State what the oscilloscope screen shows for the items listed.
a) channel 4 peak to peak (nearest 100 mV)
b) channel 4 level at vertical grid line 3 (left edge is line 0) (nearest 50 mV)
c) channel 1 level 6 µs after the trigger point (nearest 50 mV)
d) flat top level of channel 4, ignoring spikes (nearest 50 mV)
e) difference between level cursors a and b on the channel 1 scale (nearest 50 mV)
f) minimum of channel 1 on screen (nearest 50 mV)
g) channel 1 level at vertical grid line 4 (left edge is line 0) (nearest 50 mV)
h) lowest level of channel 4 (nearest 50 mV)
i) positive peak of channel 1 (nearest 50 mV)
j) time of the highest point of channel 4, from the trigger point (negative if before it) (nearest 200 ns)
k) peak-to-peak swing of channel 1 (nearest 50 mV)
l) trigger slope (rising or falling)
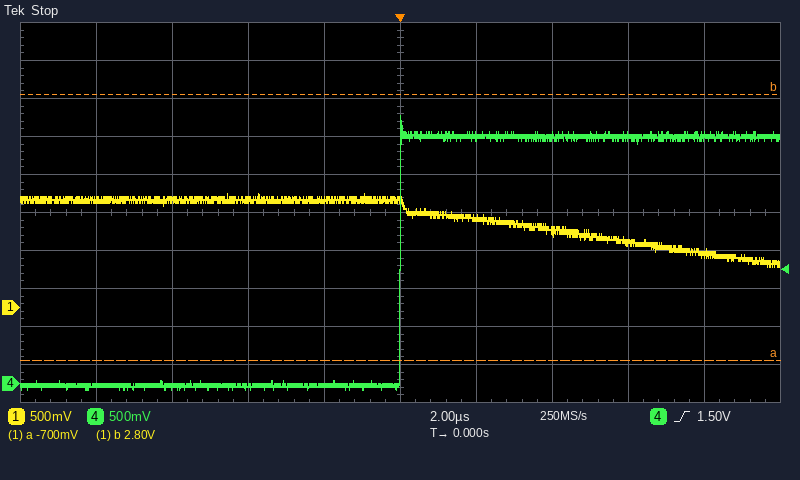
3.60 V
-50 mV
850 mV
3.25 V
3.50 V
550 mV
1.40 V
-100 mV
1.50 V
0.0 µs
950 mV
rising
